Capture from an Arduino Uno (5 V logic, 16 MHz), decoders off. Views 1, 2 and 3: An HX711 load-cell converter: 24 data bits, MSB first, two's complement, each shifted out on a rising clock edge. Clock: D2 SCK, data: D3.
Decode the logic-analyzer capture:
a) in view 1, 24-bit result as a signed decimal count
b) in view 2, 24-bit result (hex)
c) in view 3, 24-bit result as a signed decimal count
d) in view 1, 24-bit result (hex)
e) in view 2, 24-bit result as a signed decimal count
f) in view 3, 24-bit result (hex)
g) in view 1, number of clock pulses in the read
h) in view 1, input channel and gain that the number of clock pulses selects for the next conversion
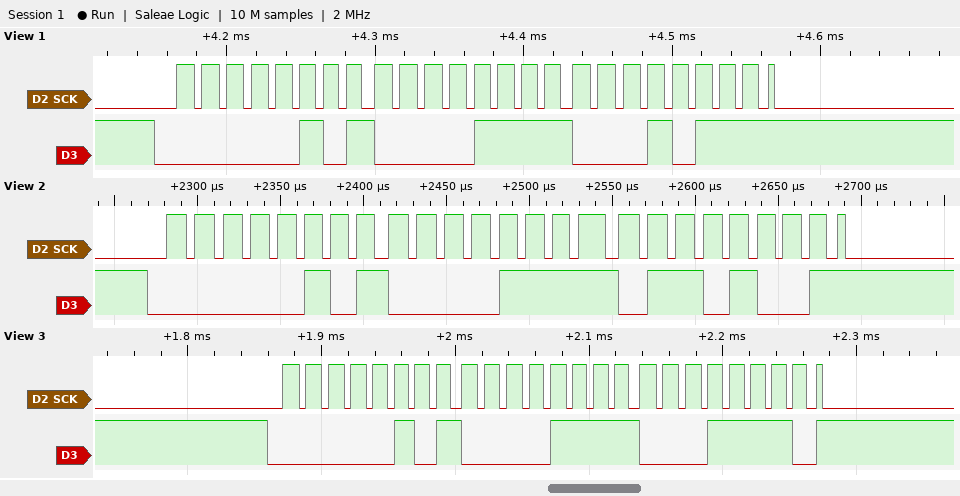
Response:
331543
0x050F69
331550
0x050F17
331625
0x050F1E
25
channel A, gain 128
